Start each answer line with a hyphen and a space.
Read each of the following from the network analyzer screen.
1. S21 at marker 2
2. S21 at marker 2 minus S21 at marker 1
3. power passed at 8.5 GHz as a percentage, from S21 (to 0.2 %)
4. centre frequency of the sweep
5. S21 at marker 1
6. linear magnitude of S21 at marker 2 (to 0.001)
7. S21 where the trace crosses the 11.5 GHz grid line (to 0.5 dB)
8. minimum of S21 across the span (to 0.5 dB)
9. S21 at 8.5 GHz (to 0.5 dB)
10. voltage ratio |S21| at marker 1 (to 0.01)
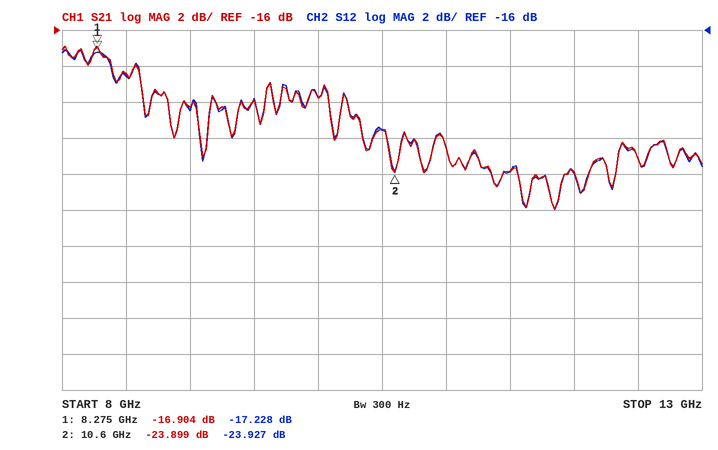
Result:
- -23.899 dB
- -6.995 dB
- 1.4 %
- 10.5 GHz
- -16.904 dB
- 0.064
- -24.0 dB
- -26.0 dB
- -18.5 dB
- 0.14
